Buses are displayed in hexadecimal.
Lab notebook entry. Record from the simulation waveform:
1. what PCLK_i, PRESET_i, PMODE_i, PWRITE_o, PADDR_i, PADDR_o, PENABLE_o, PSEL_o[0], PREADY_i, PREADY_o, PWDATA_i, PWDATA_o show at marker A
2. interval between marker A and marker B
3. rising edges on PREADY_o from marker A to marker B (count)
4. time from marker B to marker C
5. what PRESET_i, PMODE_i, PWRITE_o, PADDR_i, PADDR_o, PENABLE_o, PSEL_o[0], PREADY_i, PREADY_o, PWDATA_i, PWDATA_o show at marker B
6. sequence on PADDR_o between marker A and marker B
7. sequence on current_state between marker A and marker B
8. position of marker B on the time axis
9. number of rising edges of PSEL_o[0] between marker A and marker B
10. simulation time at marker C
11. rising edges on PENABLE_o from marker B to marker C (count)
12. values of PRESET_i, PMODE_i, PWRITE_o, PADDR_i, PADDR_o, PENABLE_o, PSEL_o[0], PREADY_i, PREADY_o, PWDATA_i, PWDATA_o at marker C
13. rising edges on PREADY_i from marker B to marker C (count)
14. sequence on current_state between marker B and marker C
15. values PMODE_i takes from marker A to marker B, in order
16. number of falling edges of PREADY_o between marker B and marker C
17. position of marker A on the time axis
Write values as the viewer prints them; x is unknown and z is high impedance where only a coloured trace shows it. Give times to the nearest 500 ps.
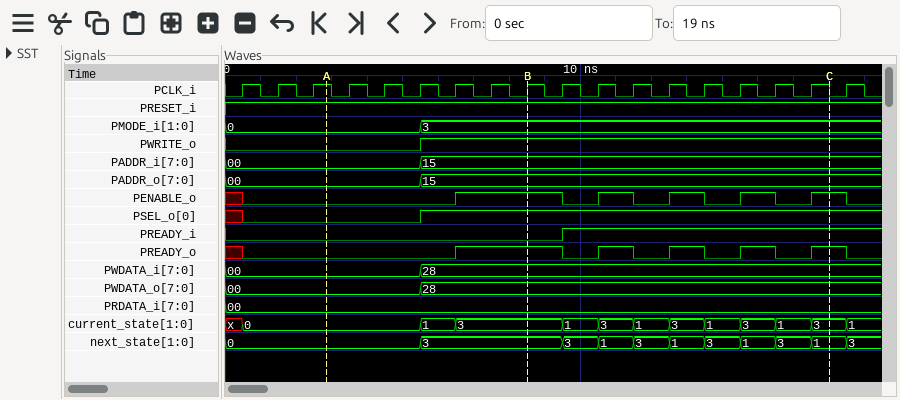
PCLK_i=1, PRESET_i=1, PMODE_i=0, PWRITE_o=0, PADDR_i=00, PADDR_o=00, PENABLE_o=0, PSEL_o[0]=0, PREADY_i=0, PREADY_o=0, PWDATA_i=00, PWDATA_o=00
5500 ps
1
8500 ps
PRESET_i=1, PMODE_i=3, PWRITE_o=1, PADDR_i=15, PADDR_o=15, PENABLE_o=1, PSEL_o[0]=1, PREADY_i=0, PREADY_o=1, PWDATA_i=28, PWDATA_o=28
00, 15
0, 1, 3
8500 ps
1
17000 ps
4
PRESET_i=1, PMODE_i=3, PWRITE_o=1, PADDR_i=15, PADDR_o=15, PENABLE_o=1, PSEL_o[0]=1, PREADY_i=1, PREADY_o=1, PWDATA_i=28, PWDATA_o=28
1
3, 1, 3, 1, 3, 1, 3, 1, 3
0, 3
4
3000 ps
